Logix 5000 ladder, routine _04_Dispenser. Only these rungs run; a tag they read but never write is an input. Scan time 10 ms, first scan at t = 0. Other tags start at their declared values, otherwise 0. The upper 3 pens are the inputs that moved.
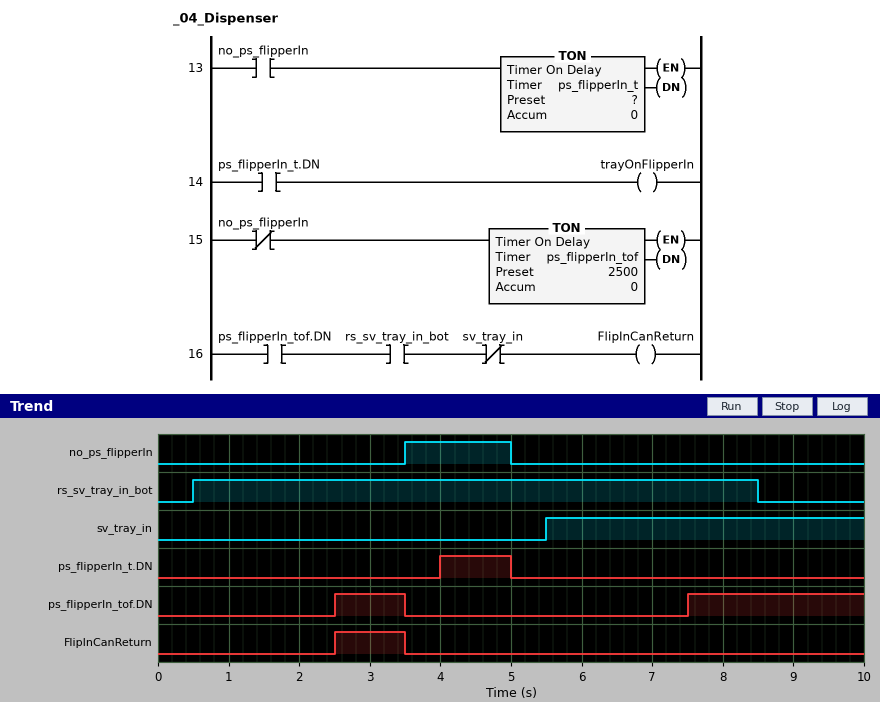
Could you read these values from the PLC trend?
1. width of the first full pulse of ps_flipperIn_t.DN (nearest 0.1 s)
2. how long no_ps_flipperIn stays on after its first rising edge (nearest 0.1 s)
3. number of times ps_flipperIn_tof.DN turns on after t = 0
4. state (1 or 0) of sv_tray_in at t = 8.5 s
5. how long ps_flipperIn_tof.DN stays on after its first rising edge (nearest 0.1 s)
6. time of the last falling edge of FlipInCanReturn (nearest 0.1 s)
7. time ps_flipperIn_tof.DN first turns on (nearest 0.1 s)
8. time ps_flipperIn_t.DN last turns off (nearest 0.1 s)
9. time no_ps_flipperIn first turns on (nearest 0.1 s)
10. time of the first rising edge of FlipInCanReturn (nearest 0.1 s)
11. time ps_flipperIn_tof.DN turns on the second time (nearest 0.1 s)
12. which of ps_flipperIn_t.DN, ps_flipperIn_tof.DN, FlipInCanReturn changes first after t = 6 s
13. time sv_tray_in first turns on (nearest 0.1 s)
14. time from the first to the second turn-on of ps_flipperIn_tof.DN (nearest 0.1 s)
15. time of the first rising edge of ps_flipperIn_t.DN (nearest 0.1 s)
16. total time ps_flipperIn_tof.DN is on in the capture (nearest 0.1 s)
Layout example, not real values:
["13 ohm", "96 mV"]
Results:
["1.0 s", "1.5 s", "2", "1", "1.0 s", "3.5 s", "2.5 s", "5.0 s", "3.5 s", "2.5 s", "7.5 s", "ps_flipperIn_tof.DN", "5.5 s", "5.0 s", "4.0 s", "3.5 s"]
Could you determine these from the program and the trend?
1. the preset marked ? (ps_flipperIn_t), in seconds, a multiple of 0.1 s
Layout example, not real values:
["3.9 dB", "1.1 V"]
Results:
["0.5 s"]
